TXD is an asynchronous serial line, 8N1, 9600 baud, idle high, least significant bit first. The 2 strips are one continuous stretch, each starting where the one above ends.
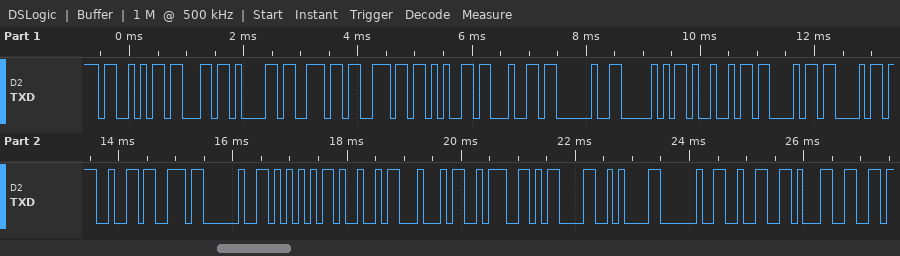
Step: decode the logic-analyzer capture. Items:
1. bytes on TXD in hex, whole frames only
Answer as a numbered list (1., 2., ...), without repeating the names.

1. 0x53 0x63 0x61 0x6E 0x6E 0x65 0x64 0x20 0x50 0x49 0x43 0x43 0x27 0x73 0x20 0x55 0x49 0x44 0x3A 0x0D 0x0A 0x20 0x32 0x31
